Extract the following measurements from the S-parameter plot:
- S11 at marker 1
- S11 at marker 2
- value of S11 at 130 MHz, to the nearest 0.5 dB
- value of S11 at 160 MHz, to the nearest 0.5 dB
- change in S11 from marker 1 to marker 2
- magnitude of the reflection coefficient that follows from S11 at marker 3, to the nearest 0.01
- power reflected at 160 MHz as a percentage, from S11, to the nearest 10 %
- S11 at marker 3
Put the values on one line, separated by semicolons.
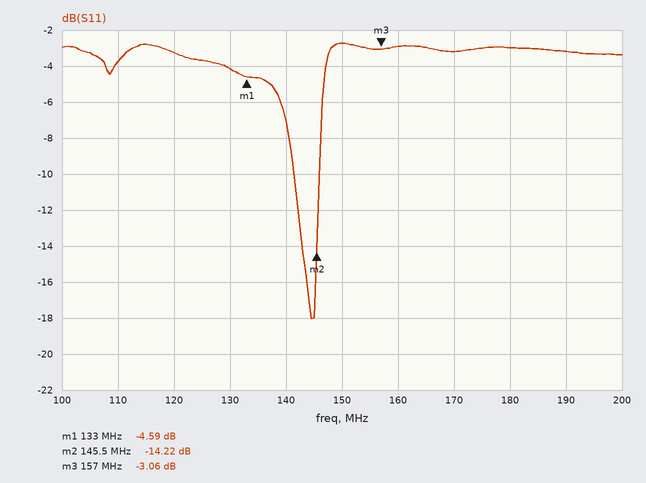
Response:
-4.59 dB; -14.22 dB; -4.0 dB; -3.0 dB; -9.63 dB; 0.70; 50 %; -3.06 dB
